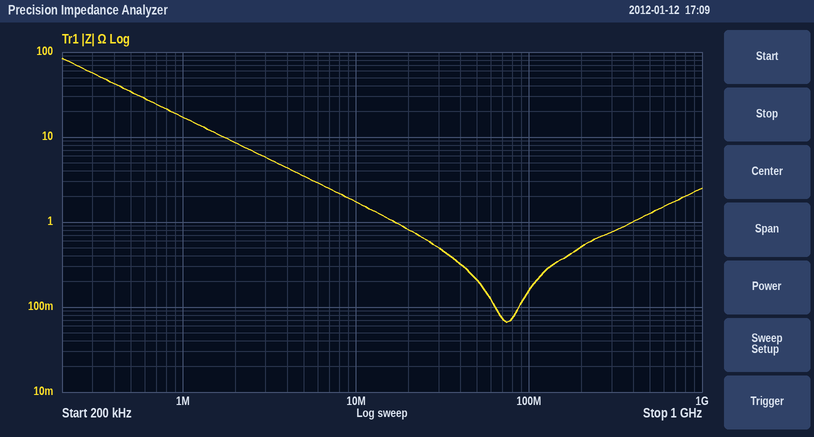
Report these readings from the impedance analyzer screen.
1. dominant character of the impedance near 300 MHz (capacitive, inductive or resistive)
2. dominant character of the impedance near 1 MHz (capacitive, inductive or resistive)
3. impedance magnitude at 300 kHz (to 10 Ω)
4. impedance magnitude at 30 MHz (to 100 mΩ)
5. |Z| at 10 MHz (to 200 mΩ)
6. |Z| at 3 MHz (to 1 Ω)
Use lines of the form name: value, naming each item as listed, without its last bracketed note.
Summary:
dominant character of the impedance near 300 MHz: inductive
dominant character of the impedance near 1 MHz: capacitive
impedance magnitude at 300 kHz: 60 Ω
impedance magnitude at 30 MHz: 500 mΩ
|Z| at 10 MHz: 1.8 Ω
|Z| at 3 MHz: 6 Ω
